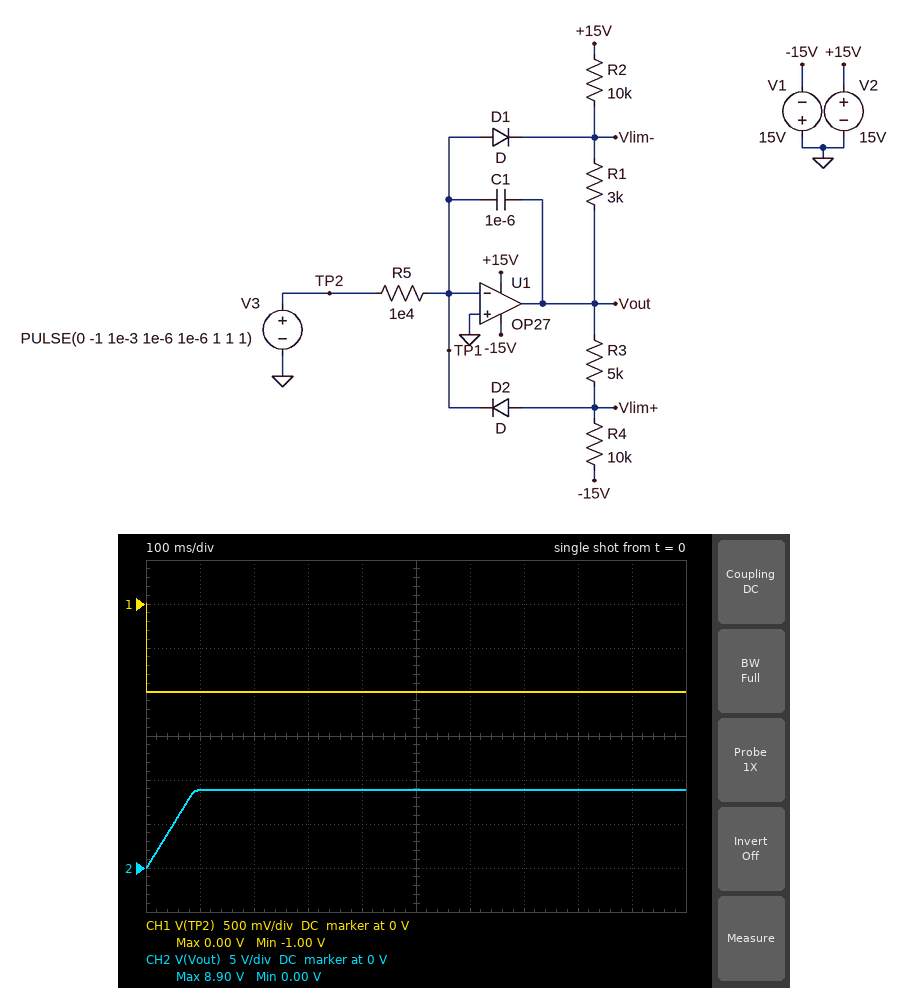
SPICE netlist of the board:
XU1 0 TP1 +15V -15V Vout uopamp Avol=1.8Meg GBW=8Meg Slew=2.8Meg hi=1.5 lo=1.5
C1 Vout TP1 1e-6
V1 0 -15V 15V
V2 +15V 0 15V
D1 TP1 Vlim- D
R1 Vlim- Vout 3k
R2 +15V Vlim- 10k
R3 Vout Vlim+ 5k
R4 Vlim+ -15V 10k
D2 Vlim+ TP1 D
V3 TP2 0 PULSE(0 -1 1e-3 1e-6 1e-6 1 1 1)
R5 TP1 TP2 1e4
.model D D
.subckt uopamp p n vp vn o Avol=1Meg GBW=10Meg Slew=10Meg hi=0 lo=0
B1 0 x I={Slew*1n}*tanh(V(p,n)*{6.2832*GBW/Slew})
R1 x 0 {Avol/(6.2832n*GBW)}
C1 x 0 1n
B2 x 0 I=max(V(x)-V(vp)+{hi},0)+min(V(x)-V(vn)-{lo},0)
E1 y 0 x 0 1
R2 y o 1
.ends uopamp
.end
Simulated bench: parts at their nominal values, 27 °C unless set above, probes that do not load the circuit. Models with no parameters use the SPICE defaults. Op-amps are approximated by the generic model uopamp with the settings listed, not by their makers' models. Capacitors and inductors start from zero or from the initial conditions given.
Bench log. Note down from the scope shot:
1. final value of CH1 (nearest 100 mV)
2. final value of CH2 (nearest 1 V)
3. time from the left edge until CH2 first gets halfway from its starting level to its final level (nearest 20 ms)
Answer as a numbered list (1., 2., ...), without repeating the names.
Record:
1. -1.0 V
2. 9 V
3. 40 ms
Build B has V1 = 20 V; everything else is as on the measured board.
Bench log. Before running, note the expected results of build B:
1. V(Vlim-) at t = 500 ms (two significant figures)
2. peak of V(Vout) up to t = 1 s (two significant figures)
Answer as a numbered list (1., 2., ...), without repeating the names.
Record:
1. 12 V
2. 11 V
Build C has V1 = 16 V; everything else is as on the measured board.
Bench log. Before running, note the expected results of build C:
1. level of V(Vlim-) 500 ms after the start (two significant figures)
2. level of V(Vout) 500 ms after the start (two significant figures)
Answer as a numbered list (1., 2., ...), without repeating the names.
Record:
1. 11 V
2. 9.4 V
